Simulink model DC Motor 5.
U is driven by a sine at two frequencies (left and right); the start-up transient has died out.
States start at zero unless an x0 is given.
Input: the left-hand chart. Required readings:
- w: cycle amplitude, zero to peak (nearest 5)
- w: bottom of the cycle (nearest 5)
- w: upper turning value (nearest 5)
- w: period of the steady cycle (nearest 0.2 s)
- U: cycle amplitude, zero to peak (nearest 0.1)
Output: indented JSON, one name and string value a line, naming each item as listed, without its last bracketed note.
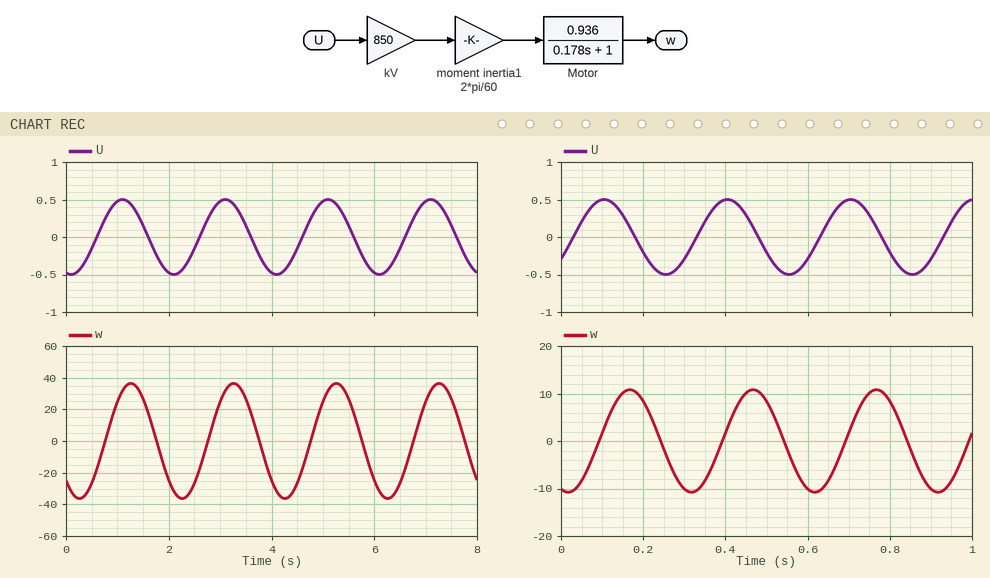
{
  "w: cycle amplitude, zero to peak": "35",
  "w: bottom of the cycle": "-35",
  "w: upper turning value": "35",
  "w: period of the steady cycle": "2.0 s",
  "U: cycle amplitude, zero to peak": "0.5"
}
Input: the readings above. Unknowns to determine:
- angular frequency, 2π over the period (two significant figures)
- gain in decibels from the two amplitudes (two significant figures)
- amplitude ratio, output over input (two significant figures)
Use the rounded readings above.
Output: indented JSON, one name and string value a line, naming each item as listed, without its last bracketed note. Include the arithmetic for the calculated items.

{
  "angular frequency, 2π over the period": "2π / 2 = 3.1 rad/s",
  "gain in decibels from the two amplitudes": "20 log10(35 / 0.5) = 37 dB",
  "amplitude ratio, output over input": "35 / 0.5 = 70"
}
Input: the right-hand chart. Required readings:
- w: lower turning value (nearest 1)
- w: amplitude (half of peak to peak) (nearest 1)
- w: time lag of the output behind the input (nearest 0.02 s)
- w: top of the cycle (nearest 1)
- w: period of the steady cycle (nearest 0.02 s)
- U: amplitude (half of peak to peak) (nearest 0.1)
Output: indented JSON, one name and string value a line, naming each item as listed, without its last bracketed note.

{
  "w: lower turning value": "-11",
  "w: amplitude (half of peak to peak)": "11",
  "w: time lag of the output behind the input": "0.06 s",
  "w: top of the cycle": "11",
  "w: period of the steady cycle": "0.30 s",
  "U: amplitude (half of peak to peak)": "0.5"
}
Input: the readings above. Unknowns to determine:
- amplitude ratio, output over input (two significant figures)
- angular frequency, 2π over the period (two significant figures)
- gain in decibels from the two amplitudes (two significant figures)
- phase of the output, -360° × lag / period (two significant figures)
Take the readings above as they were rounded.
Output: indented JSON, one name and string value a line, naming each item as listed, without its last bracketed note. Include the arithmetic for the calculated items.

{
  "amplitude ratio, output over input": "11 / 0.5 = 22",
  "angular frequency, 2π over the period": "2π / 0.3 = 21 rad/s",
  "gain in decibels from the two amplitudes": "20 log10(11 / 0.5) = 27 dB",
  "phase of the output, -360° × lag / period": "-360 × 0.06 / 0.3 = -72°"
}
